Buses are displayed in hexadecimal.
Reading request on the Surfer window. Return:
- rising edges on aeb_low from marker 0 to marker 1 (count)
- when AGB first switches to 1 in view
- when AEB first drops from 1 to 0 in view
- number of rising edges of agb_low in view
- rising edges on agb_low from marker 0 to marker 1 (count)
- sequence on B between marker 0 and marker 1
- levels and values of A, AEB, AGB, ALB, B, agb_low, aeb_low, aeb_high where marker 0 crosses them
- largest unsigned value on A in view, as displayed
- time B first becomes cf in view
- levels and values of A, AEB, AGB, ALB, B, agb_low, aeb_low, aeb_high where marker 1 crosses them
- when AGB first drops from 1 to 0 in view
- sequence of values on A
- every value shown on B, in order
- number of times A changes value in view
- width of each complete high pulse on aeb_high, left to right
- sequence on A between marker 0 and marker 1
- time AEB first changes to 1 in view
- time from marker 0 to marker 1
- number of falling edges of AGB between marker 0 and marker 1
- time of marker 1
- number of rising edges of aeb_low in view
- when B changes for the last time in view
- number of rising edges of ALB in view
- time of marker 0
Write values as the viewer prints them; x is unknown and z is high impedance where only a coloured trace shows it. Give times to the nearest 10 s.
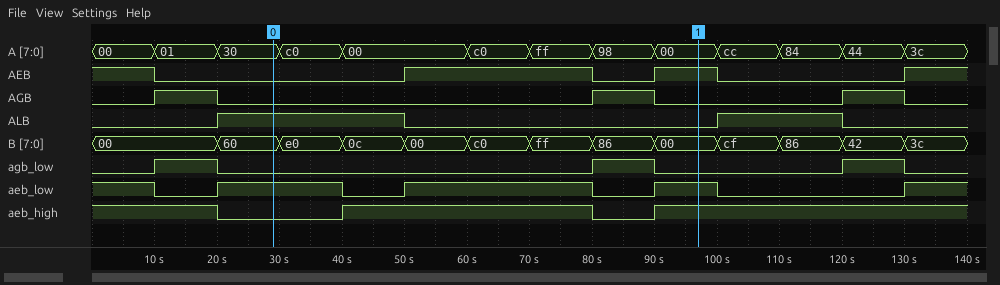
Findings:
2
10 s
10 s
3
1
60, e0, 0c, 00, c0, ff, 86, 00
A=30, AEB=0, AGB=0, ALB=1, B=60, agb_low=0, aeb_low=1, aeb_high=0
ff
100 s
A=00, AEB=1, AGB=0, ALB=0, B=00, agb_low=0, aeb_low=1, aeb_high=1
20 s
00, 01, 30, c0, 00, c0, ff, 98, 00, cc, 84, 44, 3c
00, 60, e0, 0c, 00, c0, ff, 86, 00, cf, 86, 42, 3c
12
40 s
30, c0, 00, c0, ff, 98, 00
50 s
70 s
1
100 s
4
130 s
2
30 s
